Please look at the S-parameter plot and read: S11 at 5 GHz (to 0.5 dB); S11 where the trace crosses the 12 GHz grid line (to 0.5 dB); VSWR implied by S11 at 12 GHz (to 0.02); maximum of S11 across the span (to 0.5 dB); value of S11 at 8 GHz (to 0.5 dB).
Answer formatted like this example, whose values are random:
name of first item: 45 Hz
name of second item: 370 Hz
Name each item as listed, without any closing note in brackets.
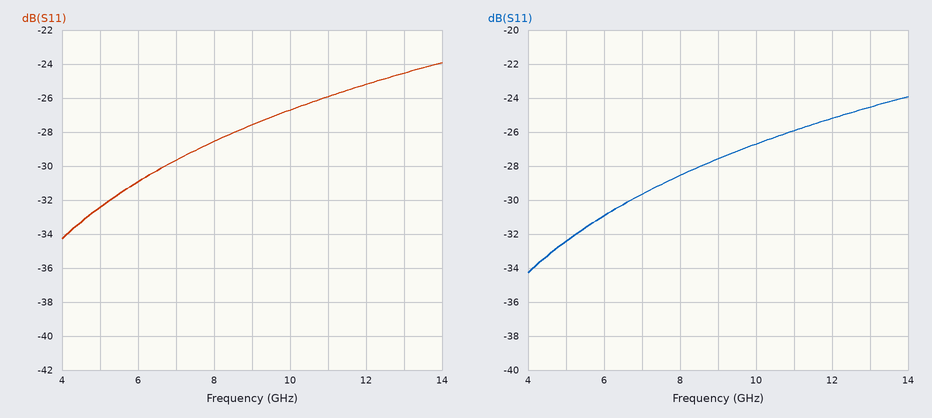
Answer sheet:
S11 at 5 GHz: -32.5 dB
S11 where the trace crosses the 12 GHz grid line: -25.0 dB
VSWR implied by S11 at 12 GHz: 1.12
maximum of S11 across the span: -24.0 dB
value of S11 at 8 GHz: -28.5 dB
